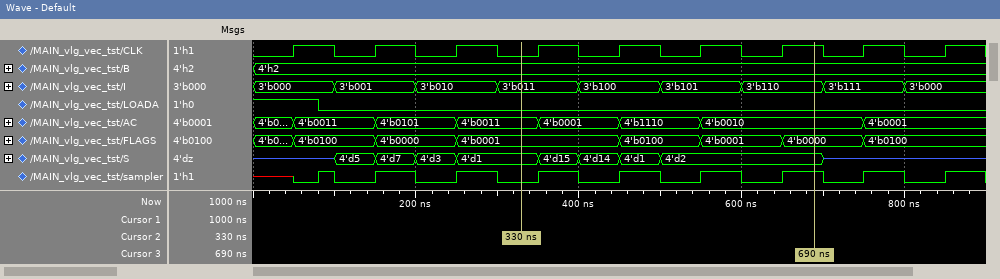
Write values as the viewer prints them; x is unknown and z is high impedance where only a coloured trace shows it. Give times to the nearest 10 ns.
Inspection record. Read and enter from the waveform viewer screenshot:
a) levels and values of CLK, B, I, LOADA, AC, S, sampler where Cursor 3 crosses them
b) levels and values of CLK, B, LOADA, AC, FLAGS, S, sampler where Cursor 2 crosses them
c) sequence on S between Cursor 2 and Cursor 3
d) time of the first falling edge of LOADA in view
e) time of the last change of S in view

CLK=1, B=4'h2, I=3'b110, LOADA=0, AC=4'b0010, S=4'd2, sampler=1
CLK=0, B=4'h2, LOADA=0, AC=4'b0011, FLAGS=4'b0001, S=4'd1, sampler=0
4'd1, 4'd15, 4'd14, 4'd1, 4'd2
80 ns
700 ns
